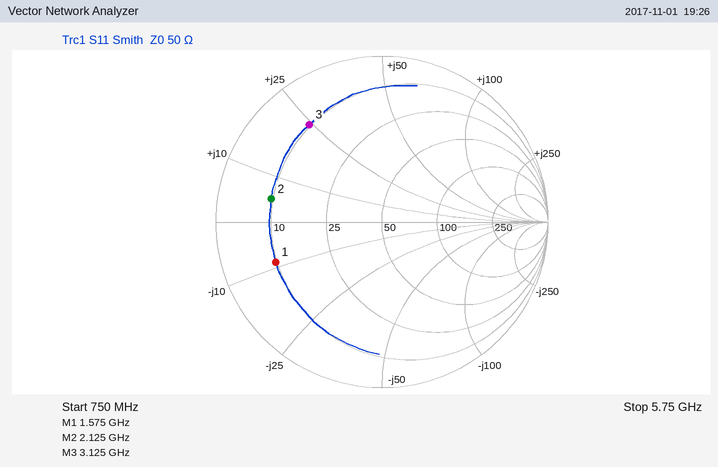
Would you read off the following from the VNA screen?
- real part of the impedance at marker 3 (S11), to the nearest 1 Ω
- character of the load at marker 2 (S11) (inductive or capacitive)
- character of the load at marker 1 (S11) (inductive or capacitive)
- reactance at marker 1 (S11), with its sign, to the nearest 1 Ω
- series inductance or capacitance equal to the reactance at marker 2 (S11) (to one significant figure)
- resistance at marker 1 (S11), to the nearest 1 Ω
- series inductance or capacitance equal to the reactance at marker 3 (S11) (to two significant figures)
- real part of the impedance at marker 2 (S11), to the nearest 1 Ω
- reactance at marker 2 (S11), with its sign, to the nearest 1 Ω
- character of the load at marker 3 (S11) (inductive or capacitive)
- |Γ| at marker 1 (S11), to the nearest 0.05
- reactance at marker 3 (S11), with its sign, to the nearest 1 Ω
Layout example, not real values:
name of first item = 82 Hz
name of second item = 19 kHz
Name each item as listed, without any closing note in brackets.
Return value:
real part of the impedance at marker 3 (S11), to the nearest 1 Ω = 10 Ω
character of the load at marker 2 (S11) = inductive
character of the load at marker 1 (S11) = capacitive
reactance at marker 1 (S11), with its sign, to the nearest 1 Ω = -9 Ω
series inductance or capacitance equal to the reactance at marker 2 (S11) = 400 pH
resistance at marker 1 (S11), to the nearest 1 Ω = 10 Ω
series inductance or capacitance equal to the reactance at marker 3 (S11) = 1.2 nH
real part of the impedance at marker 2 (S11), to the nearest 1 Ω = 10 Ω
reactance at marker 2 (S11), with its sign, to the nearest 1 Ω = +5 Ω
character of the load at marker 3 (S11) = inductive
|Γ| at marker 1 (S11), to the nearest 0.05 = 0.70
reactance at marker 3 (S11), with its sign, to the nearest 1 Ω = +24 Ω
